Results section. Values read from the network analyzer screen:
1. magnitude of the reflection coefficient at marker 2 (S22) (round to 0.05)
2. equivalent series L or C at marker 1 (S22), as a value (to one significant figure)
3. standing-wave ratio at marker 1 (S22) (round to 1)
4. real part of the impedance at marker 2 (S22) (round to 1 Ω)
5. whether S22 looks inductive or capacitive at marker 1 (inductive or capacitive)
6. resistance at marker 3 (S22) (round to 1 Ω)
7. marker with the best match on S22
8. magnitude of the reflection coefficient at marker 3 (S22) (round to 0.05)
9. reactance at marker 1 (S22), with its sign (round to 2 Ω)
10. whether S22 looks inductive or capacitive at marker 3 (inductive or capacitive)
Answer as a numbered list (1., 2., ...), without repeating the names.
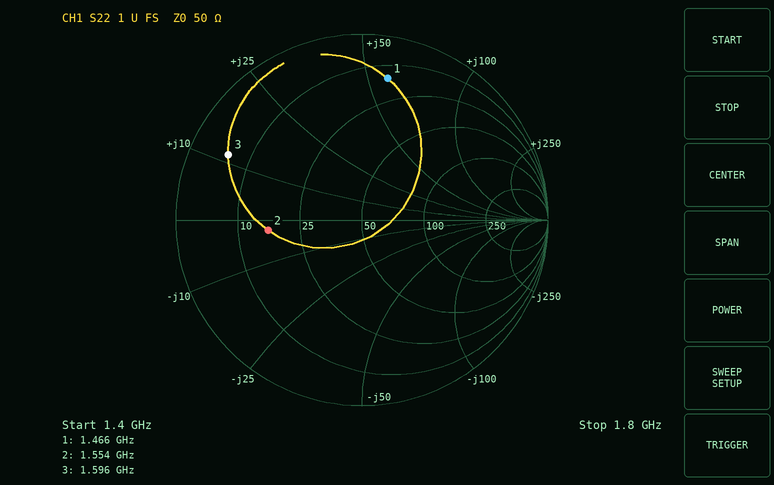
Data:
1. 0.50
2. 6 nH
3. 8
4. 16 Ω
5. inductive
6. 6 Ω
7. marker 2
8. 0.80
9. +58 Ω
10. inductive
